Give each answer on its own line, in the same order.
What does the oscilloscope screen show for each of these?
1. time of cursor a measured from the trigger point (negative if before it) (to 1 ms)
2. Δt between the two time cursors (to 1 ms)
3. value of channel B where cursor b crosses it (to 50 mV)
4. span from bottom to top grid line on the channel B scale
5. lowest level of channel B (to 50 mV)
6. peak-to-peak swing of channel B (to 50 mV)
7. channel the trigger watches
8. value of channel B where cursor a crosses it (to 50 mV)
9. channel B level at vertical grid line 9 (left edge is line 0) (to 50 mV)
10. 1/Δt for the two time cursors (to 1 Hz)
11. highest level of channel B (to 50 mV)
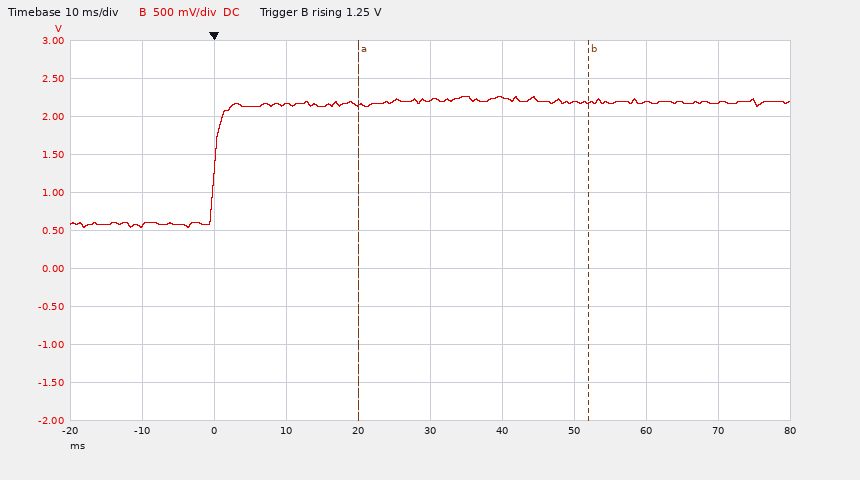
+20 ms
32 ms
2.20 V
5 V
550 mV
1.70 V
channel B
2.15 V
2.20 V
31 Hz
2.25 V
